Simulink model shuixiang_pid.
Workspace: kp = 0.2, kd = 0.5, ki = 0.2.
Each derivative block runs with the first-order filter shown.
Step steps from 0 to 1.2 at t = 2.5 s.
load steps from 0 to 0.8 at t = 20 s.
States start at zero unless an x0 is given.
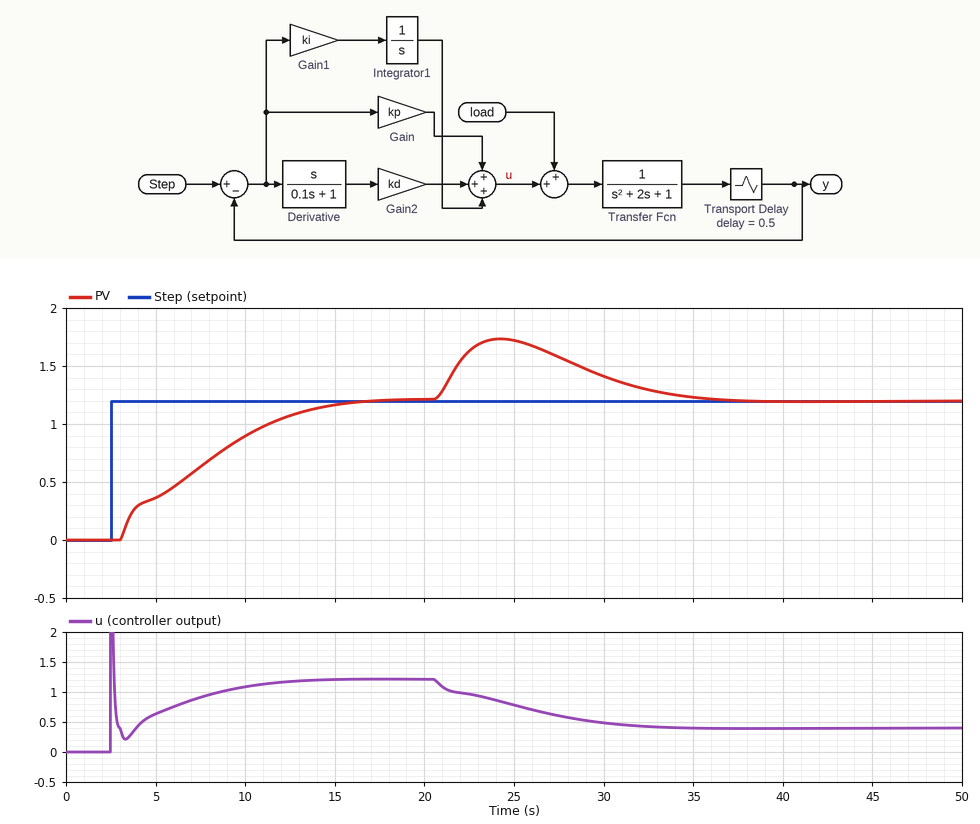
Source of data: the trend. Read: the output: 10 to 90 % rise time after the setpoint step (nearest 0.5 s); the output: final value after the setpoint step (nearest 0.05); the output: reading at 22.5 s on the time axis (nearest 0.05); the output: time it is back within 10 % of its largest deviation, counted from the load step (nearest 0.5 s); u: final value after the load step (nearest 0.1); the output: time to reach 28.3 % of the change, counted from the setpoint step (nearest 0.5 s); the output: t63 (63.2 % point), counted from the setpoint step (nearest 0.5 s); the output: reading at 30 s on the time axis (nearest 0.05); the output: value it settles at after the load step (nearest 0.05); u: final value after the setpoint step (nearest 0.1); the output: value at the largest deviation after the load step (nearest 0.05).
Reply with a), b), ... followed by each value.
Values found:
a) 9.5 s
b) 1.20
c) 1.65
d) 14.0 s
e) 0.4
f) 2.0 s
g) 6.0 s
h) 1.40
i) 1.20
j) 1.2
k) 1.75
